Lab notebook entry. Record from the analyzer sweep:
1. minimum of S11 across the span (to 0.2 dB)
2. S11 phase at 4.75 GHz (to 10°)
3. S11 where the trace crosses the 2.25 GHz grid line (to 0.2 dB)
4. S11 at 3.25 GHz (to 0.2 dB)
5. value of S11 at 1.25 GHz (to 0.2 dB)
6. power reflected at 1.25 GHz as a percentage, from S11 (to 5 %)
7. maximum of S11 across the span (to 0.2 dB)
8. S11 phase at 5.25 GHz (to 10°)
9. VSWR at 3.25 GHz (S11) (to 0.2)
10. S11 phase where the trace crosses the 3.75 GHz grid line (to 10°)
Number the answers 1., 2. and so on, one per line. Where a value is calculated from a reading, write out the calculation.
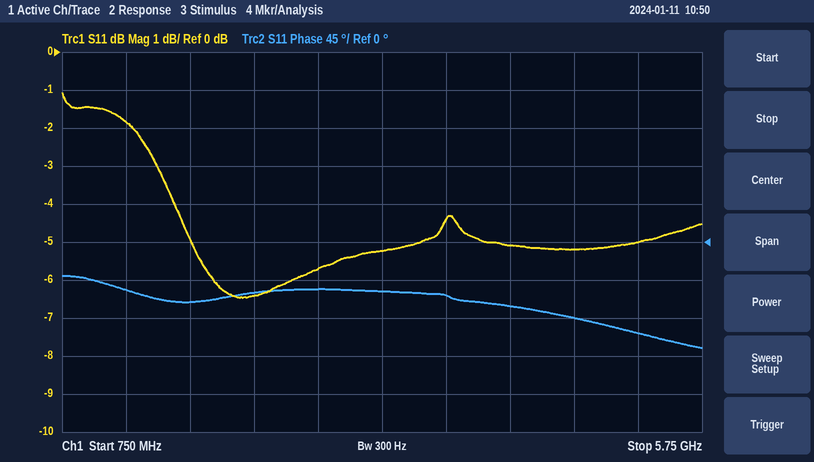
1. -6.4 dB
2. -90°
3. -6.4 dB
4. -5.2 dB
5. -1.8 dB
6. 10^(-1.8/10) ≈ 66.1 %, so 65 % to the nearest 5 %
7. -1.0 dB
8. -110°
9. |Γ| = 10^(-5.2/20) = 0.5495; VSWR = (1 + 0.5495)/(1 − 0.5495) ≈ 3.4
10. -60°
